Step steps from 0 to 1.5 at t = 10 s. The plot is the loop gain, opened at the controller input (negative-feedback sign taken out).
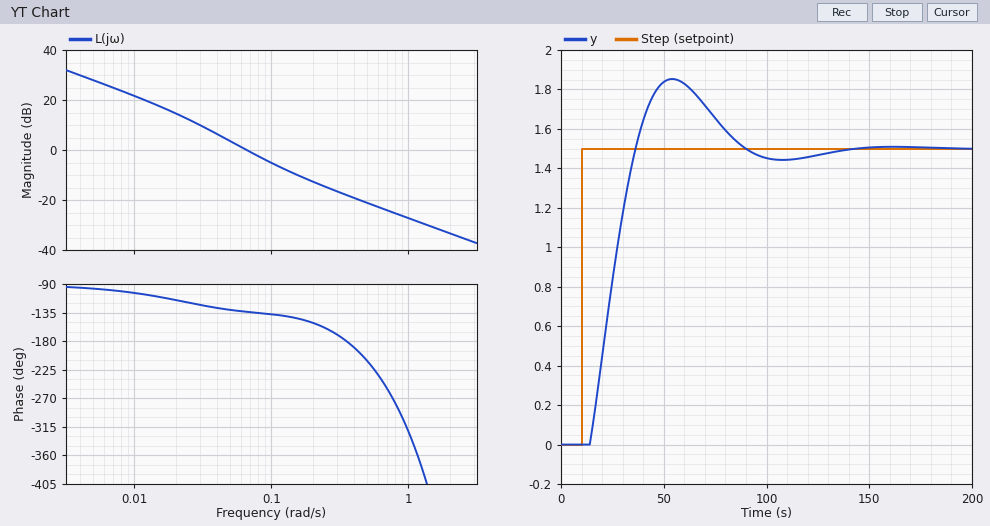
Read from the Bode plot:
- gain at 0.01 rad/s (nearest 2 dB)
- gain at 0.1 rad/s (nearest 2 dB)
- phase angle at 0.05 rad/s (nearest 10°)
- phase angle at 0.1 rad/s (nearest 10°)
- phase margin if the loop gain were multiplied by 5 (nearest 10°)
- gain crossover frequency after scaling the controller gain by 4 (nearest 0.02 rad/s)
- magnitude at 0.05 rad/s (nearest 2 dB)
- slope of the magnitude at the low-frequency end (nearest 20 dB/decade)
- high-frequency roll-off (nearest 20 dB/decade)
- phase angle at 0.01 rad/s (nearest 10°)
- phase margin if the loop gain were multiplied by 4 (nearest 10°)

22 dB
-6 dB
-130°
-140°
20°
0.18 rad/s
4 dB
-20 dB/decade
-20 dB/decade
-100°
30°
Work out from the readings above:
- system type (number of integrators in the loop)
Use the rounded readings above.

1
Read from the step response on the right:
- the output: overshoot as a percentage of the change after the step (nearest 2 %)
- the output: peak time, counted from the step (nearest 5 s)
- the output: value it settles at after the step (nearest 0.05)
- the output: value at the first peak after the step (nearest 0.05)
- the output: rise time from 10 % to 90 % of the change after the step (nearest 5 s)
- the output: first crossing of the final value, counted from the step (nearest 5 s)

24 %
45 s
1.50
1.85
15 s
25 s
